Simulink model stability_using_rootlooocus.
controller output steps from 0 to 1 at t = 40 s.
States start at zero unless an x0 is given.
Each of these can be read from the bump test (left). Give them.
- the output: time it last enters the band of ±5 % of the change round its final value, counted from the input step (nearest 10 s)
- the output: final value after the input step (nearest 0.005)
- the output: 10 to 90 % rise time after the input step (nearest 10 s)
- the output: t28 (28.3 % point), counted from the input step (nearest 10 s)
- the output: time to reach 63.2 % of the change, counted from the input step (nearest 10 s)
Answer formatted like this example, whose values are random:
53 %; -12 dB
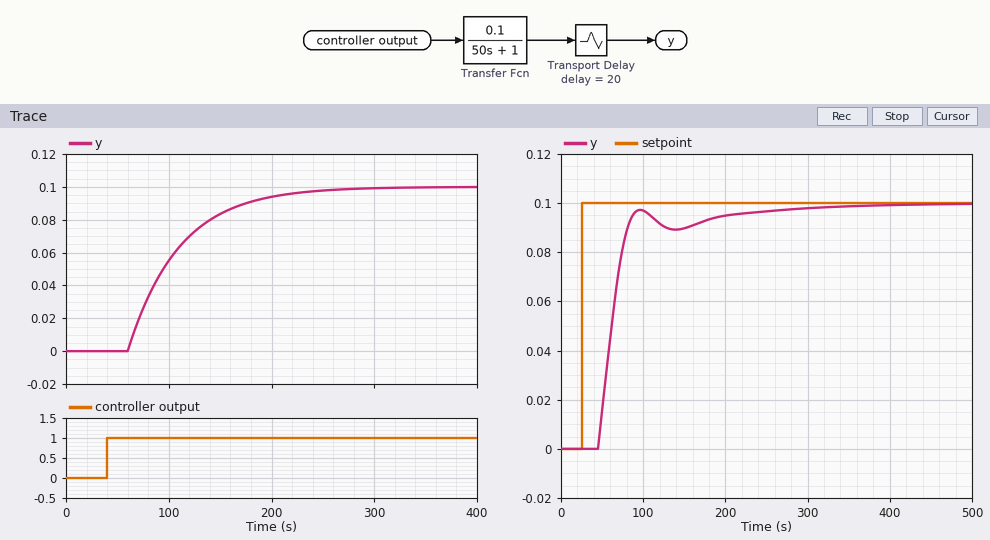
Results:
170 s; 0.100; 110 s; 40 s; 70 s
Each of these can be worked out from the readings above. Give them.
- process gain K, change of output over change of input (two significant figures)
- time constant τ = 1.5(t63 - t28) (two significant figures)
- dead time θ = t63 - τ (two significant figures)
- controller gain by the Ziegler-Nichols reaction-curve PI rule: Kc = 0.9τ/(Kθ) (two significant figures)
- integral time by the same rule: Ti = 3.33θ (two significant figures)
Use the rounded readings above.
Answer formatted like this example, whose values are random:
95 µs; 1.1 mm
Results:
0.10; 45 s; 25 s; 16; 83 s
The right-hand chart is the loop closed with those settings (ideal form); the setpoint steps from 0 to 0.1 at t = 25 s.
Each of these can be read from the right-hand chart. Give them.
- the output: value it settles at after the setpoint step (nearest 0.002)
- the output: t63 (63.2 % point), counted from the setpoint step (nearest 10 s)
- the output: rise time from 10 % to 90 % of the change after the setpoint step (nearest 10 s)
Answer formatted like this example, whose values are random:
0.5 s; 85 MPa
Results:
0.100; 40 s; 30 s
